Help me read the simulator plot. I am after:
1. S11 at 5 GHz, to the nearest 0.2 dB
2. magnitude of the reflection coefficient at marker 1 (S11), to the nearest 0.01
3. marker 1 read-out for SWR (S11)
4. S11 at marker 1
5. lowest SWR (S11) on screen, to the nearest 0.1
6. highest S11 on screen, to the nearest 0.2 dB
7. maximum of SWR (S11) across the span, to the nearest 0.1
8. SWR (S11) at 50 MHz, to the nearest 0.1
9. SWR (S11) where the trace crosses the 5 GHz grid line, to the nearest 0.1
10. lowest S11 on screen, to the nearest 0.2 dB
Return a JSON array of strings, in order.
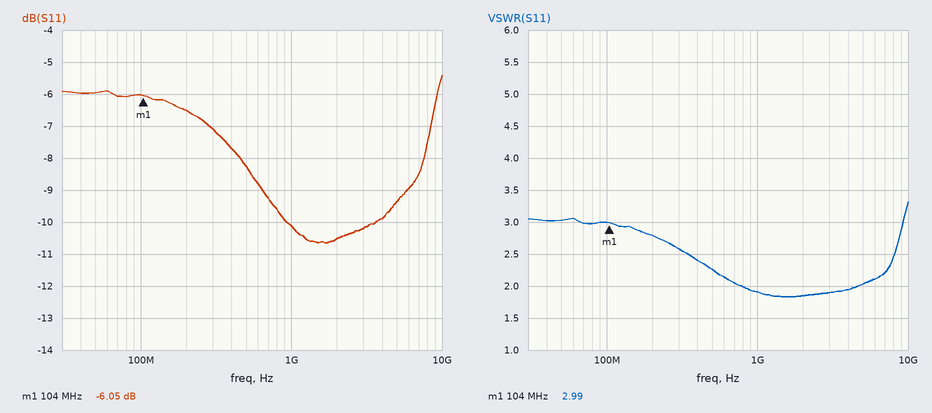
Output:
["-9.4 dB", "0.50", "2.99", "-6.05 dB", "1.8", "-5.4 dB", "3.3", "3.0", "2.0", "-10.6 dB"]
